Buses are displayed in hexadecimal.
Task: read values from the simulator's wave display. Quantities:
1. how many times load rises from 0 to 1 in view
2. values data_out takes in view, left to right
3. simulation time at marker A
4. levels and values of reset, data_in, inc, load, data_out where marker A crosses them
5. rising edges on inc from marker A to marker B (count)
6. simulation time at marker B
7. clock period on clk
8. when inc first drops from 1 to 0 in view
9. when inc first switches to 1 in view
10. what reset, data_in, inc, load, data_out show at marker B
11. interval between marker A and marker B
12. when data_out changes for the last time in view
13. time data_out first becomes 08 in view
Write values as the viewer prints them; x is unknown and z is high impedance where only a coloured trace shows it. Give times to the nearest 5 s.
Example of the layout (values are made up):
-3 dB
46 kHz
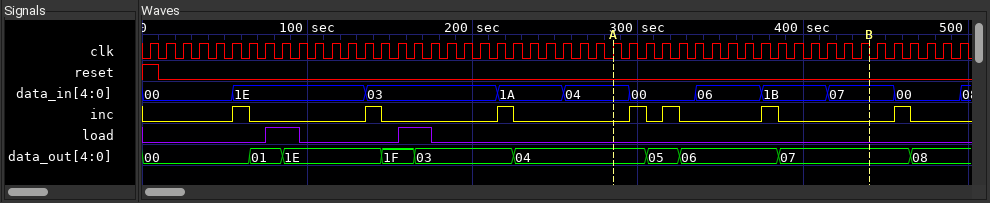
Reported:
2
00, 01, 1E, 1F, 03, 04, 05, 06, 07, 08
285 s
reset=0, data_in=04, inc=0, load=0, data_out=04
3
440 s
10 s
65 s
55 s
reset=0, data_in=07, inc=0, load=0, data_out=07
155 s
465 s
465 s
